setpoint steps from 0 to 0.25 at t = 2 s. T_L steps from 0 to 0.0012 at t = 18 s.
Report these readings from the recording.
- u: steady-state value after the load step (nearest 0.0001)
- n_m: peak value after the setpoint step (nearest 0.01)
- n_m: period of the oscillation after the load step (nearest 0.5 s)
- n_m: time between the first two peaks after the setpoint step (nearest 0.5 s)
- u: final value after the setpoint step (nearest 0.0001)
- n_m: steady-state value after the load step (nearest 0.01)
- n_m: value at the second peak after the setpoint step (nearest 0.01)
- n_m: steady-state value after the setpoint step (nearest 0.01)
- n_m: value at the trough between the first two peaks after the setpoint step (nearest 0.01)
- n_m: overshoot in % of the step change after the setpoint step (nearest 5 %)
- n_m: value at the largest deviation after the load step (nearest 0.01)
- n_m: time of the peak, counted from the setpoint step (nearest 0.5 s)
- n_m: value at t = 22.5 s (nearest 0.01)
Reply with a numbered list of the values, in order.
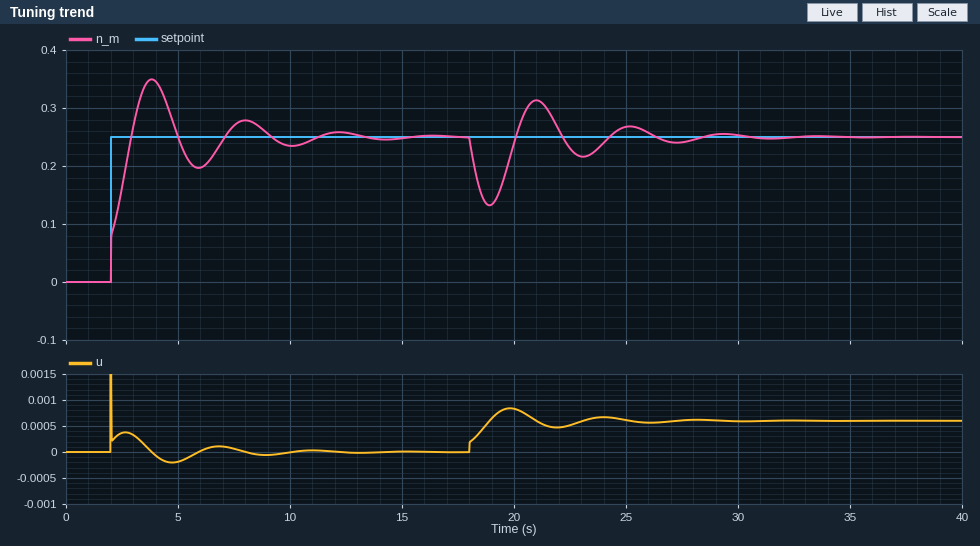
1. 0.0006
2. 0.35
3. 4.0 s
4. 4.0 s
5. 0.0000
6. 0.25
7. 0.28
8. 0.25
9. 0.20
10. 40 %
11. 0.13
12. 2.0 s
13. 0.23
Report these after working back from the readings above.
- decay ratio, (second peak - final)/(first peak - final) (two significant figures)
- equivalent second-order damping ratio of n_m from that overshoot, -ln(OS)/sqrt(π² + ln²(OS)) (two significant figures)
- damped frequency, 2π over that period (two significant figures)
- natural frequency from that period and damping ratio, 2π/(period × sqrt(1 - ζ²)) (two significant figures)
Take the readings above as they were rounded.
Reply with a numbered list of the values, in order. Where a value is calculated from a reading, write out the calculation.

1. (0.28 - 0.25) / (0.35 - 0.25) = 0.30
2. ln(0.4) = -0.916; 0.916 / sqrt(9.870 + 0.840) = 0.28
3. 2π / 4 = 1.6 rad/s
4. 2π / (4 × sqrt(1 - 0.28²)) = 1.6 rad/s
